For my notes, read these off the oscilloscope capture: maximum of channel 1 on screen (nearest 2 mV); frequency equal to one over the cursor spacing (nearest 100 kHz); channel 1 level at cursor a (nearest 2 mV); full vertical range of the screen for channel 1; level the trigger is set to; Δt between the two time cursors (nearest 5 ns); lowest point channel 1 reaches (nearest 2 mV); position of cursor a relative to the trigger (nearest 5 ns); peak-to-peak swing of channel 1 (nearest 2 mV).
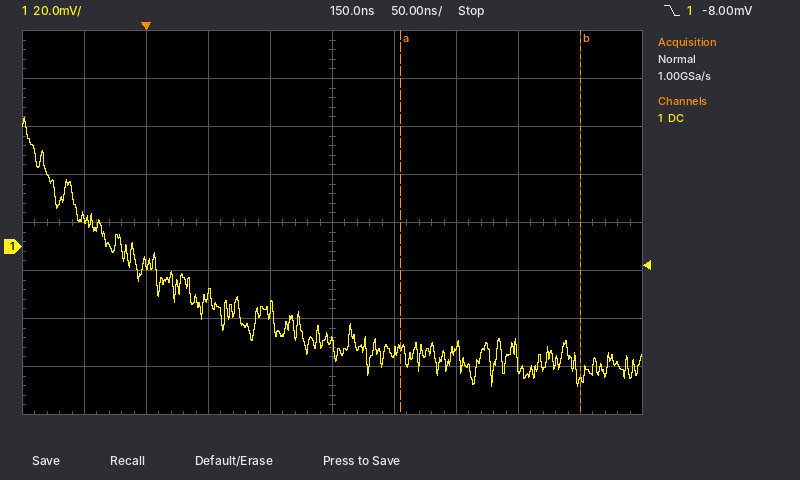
54 mV
6.9 MHz
-42 mV
160 mV
-8.00 mV
145 ns
-58 mV
+205 ns
112 mV
